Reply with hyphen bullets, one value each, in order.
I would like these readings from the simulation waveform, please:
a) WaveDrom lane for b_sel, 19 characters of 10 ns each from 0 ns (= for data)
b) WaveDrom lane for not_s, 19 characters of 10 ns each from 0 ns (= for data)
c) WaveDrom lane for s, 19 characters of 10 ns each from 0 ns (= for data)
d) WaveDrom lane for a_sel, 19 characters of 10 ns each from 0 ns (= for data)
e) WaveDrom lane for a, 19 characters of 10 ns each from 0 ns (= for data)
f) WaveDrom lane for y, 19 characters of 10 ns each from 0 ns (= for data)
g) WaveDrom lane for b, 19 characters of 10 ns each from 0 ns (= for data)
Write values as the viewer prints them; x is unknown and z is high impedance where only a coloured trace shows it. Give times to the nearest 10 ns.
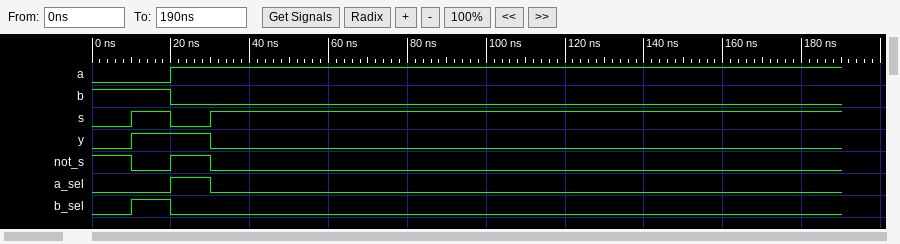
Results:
- {name: 'b_sel', wave: '010................'}
- {name: 'not_s', wave: '1010...............'}
- {name: 's', wave: '0101...............'}
- {name: 'a_sel', wave: '0.10...............'}
- {name: 'a', wave: '0.1................'}
- {name: 'y', wave: '01.0...............'}
- {name: 'b', wave: '1.0................'}
